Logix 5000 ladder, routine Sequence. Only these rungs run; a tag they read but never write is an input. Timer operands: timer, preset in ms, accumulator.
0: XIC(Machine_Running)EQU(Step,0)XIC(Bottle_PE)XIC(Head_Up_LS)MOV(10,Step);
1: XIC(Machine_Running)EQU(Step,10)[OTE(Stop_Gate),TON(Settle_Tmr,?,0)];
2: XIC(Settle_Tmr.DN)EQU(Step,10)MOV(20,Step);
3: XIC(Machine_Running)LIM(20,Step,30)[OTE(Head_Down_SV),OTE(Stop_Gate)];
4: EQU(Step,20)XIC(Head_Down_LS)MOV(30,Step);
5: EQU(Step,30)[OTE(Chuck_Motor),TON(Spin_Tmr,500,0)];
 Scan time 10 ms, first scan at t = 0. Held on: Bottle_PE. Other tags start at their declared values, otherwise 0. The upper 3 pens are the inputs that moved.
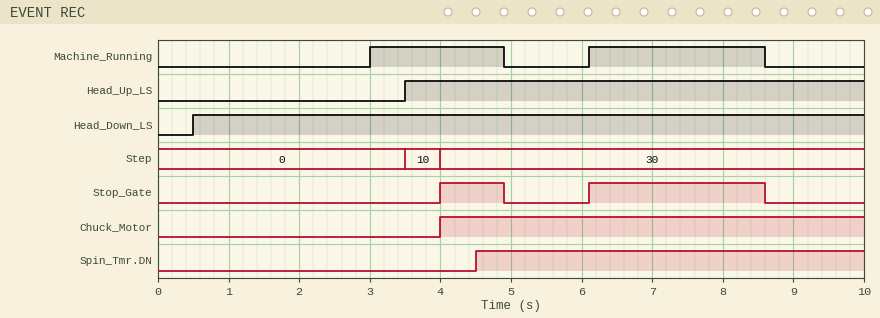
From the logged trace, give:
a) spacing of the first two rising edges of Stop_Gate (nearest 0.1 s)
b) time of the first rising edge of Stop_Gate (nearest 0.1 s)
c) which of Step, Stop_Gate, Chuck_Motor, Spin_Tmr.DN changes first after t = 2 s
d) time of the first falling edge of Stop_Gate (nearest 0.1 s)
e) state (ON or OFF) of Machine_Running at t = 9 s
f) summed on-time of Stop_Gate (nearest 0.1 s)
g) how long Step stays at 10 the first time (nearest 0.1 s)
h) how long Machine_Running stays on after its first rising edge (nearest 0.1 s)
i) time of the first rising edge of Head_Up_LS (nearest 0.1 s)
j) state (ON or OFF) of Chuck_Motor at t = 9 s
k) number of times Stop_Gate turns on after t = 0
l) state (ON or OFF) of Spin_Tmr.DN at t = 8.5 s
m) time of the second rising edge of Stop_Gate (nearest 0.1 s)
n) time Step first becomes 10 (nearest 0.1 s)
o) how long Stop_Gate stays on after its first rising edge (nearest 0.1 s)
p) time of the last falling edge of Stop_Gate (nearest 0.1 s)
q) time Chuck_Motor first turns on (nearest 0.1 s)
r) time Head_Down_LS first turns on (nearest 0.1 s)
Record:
2.1 s
4.0 s
Step
4.9 s
OFF
3.4 s
0.5 s
1.9 s
3.5 s
ON
2
ON
6.1 s
3.5 s
0.9 s
8.6 s
4.0 s
0.5 s
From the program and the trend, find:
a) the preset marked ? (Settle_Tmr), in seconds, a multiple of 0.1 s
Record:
0.5 s
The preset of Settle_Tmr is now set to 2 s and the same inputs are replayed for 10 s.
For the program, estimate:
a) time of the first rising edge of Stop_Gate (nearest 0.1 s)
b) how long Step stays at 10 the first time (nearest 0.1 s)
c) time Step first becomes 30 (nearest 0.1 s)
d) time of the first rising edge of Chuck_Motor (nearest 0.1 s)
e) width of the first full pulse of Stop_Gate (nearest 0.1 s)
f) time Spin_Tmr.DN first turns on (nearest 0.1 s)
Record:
8.1 s
4.6 s
8.1 s
8.1 s
0.5 s
8.6 s
